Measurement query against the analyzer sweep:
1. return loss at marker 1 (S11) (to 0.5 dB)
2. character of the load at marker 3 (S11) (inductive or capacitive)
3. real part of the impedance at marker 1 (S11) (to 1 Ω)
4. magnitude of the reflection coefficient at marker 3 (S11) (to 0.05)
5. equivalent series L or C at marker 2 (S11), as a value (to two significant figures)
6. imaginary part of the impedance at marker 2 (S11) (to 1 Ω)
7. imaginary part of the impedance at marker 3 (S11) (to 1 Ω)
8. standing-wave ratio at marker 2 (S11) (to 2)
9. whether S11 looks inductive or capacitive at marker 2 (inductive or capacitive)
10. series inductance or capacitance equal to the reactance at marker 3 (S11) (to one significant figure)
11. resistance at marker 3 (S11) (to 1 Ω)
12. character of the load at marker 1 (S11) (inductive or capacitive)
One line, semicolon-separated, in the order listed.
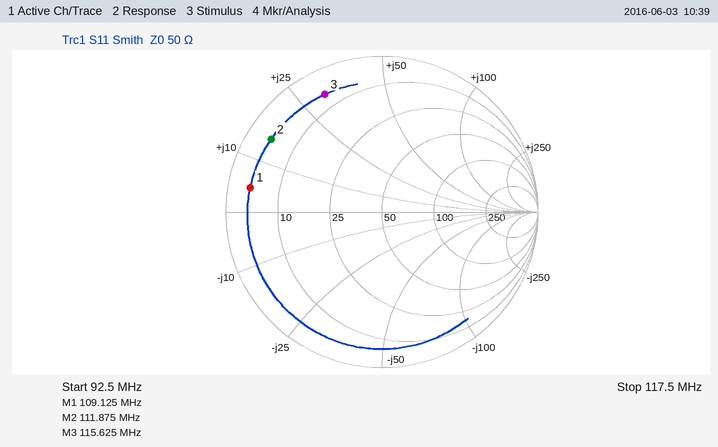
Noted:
1.5 dB; inductive; 4 Ω; 0.85; 21 nH; +15 Ω; +31 Ω; 12; inductive; 40 nH; 6 Ω; inductive
